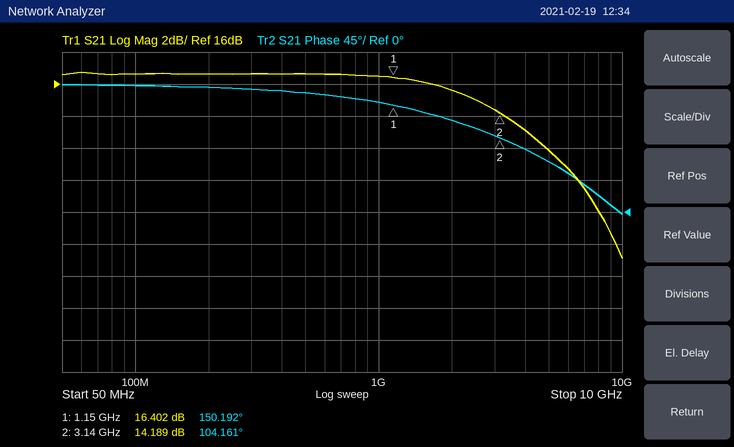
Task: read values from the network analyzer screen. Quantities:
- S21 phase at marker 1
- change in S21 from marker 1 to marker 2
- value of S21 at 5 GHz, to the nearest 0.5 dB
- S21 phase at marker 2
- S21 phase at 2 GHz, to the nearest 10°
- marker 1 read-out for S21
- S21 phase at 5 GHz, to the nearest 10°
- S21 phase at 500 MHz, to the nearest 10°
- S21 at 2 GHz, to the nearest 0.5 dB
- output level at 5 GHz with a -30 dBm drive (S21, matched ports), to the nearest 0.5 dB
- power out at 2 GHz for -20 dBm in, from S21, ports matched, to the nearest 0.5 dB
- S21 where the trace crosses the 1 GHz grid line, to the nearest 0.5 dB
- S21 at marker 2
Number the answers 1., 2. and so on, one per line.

1. 150.192°
2. -2.213 dB
3. 12.0 dB
4. 104.161°
5. 130°
6. 16.402 dB
7. 70°
8. 170°
9. 15.5 dB
10. -18.0 dBm
11. -4.5 dBm
12. 16.5 dB
13. 14.189 dB
